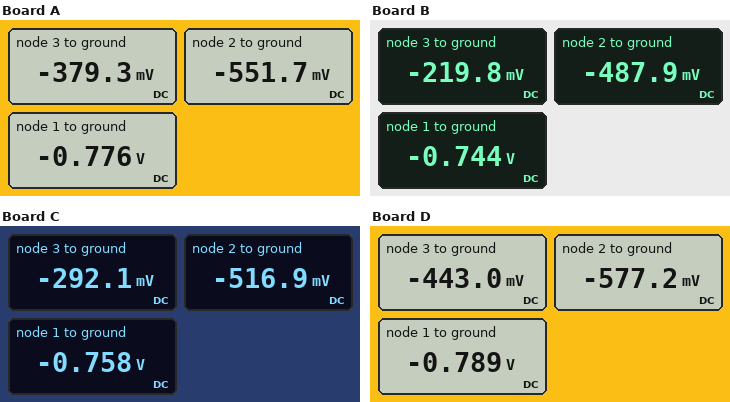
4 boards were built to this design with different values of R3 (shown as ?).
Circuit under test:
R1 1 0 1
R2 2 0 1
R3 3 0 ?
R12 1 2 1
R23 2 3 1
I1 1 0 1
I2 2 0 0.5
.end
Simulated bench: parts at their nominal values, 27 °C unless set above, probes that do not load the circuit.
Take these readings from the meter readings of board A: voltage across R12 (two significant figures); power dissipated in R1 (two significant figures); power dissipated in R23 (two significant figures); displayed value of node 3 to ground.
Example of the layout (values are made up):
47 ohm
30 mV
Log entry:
220 mV
600 mW
30 mW
-379.3 mV
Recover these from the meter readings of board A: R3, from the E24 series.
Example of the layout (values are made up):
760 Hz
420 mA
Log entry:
2.2 Ω
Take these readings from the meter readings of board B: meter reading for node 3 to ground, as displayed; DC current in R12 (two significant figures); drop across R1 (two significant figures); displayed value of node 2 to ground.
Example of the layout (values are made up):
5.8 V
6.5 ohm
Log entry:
-219.8 mV
260 mA
740 mV
-487.9 mV
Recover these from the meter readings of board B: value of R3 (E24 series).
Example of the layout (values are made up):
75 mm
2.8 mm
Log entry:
0.82 Ω
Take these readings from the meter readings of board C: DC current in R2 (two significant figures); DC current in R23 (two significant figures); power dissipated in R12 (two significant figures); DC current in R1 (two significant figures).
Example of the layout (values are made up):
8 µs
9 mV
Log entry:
520 mA
220 mA
58 mW
760 mA
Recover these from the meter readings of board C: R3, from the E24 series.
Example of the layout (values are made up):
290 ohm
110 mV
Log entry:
1.3 Ω
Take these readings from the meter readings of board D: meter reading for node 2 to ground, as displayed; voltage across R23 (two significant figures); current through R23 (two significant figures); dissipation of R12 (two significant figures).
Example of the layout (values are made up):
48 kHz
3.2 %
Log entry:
-577.2 mV
130 mV
130 mA
45 mW
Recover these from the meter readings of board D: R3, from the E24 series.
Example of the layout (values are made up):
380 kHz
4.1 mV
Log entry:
3.3 Ω
